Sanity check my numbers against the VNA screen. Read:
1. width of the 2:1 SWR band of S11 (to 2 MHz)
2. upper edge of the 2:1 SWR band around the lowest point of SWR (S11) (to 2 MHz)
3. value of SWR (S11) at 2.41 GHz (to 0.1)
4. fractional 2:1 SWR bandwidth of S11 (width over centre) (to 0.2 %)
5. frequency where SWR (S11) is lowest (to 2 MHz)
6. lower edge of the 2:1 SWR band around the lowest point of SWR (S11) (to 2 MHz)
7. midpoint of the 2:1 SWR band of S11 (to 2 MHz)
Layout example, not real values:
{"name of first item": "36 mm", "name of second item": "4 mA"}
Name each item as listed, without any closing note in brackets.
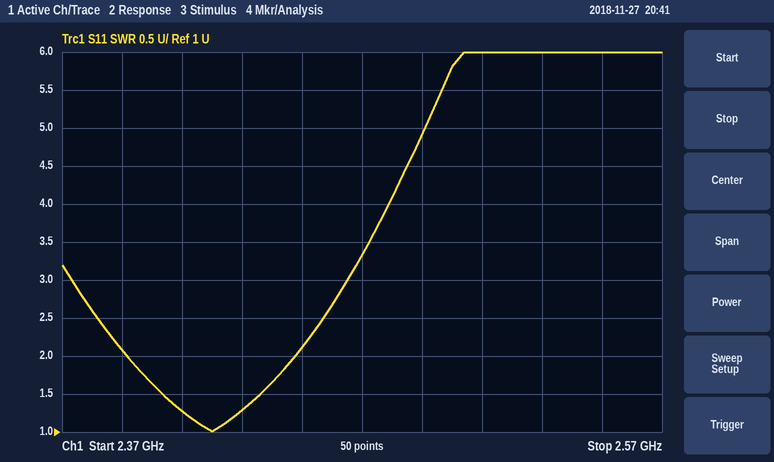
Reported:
{"width of the 2:1 SWR band of S11": "56 MHz", "upper edge of the 2:1 SWR band around the lowest point of SWR (S11)": "2.448 GHz", "value of SWR (S11) at 2.41 GHz": "1.3", "fractional 2:1 SWR bandwidth of S11 (width over centre)": "2.4 %", "frequency where SWR (S11) is lowest": "2.420 GHz", "lower edge of the 2:1 SWR band around the lowest point of SWR (S11)": "2.392 GHz", "midpoint of the 2:1 SWR band of S11": "2.420 GHz"}
